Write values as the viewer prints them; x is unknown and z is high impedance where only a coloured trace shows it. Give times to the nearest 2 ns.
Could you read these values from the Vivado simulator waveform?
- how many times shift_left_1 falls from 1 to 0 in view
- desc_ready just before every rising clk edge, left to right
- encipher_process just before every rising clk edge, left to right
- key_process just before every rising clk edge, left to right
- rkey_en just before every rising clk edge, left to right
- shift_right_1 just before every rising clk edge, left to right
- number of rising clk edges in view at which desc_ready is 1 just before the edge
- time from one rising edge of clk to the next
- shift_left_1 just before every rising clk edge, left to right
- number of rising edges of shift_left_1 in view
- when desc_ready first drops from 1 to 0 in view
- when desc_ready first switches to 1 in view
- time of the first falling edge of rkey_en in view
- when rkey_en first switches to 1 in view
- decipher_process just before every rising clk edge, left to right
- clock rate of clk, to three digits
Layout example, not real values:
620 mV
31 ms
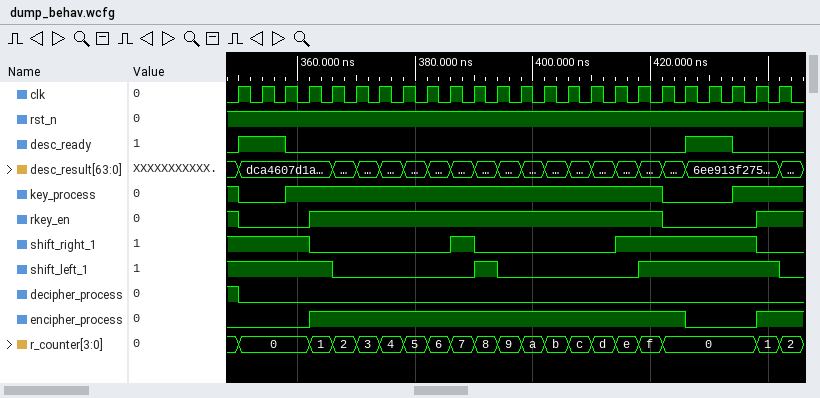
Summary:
3
0 1 1 0 0 0 0 0 0 0 0 0 0 0 0 0 0 0 0 0 1 1 0 0
0 0 0 0 1 1 1 1 1 1 1 1 1 1 1 1 1 1 1 1 0 0 0 1
1 0 0 1 1 1 1 1 1 1 1 1 1 1 1 1 1 1 1 0 0 0 1 1
1 0 0 0 1 1 1 1 1 1 1 1 1 1 1 1 1 1 1 0 0 0 0 1
1 1 1 1 0 0 0 0 0 0 1 0 0 0 0 0 0 1 1 1 1 1 1 0
4
4 ns
1 1 1 1 1 0 0 0 0 0 0 1 0 0 0 0 0 0 1 1 1 1 1 1
2
358 ns
350 ns
350 ns
362 ns
1 0 0 0 0 0 0 0 0 0 0 0 0 0 0 0 0 0 0 0 0 0 0 0
250 MHz
